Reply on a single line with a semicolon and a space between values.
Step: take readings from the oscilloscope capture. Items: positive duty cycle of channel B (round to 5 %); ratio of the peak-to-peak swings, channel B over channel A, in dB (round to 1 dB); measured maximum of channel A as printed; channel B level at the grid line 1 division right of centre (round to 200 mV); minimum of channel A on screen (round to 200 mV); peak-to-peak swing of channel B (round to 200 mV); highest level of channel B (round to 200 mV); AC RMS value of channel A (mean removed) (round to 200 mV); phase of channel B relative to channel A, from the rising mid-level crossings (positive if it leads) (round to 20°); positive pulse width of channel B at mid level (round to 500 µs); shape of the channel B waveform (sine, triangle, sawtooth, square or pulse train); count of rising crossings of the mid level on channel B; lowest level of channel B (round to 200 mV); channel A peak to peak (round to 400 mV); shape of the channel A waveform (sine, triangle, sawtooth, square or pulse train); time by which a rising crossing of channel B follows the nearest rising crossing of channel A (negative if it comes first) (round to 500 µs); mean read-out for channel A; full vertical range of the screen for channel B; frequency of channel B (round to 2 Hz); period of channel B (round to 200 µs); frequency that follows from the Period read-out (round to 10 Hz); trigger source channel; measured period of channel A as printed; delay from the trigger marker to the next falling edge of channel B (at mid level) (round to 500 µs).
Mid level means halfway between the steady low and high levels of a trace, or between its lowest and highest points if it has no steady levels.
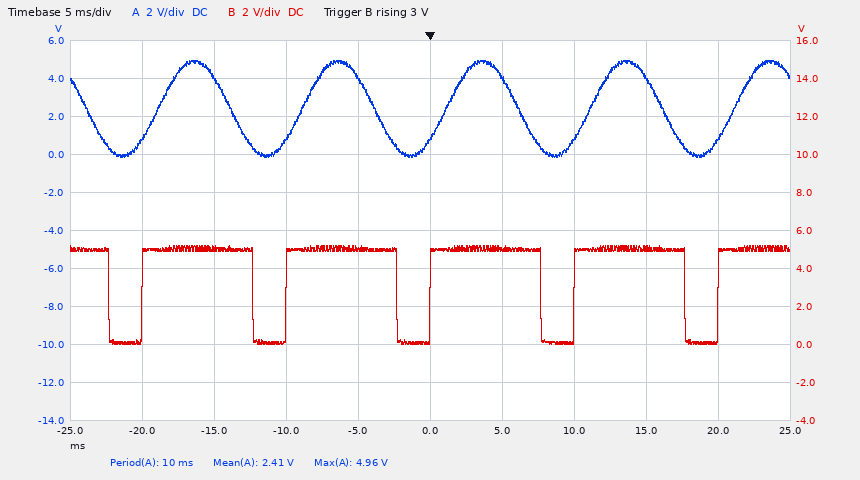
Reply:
75 %; 0 dB; 4.96 V; 5.0 V; -200 mV; 5.2 V; 5.2 V; 1.8 V; +40°; 7.5 ms; pulse train; 5; 0.0 V; 5.2 V; sine; -1.0 ms; 2.41 V; 20 V; 100 Hz; 10.0 ms; 100 Hz; channel B; 10 ms; 7.5 ms
